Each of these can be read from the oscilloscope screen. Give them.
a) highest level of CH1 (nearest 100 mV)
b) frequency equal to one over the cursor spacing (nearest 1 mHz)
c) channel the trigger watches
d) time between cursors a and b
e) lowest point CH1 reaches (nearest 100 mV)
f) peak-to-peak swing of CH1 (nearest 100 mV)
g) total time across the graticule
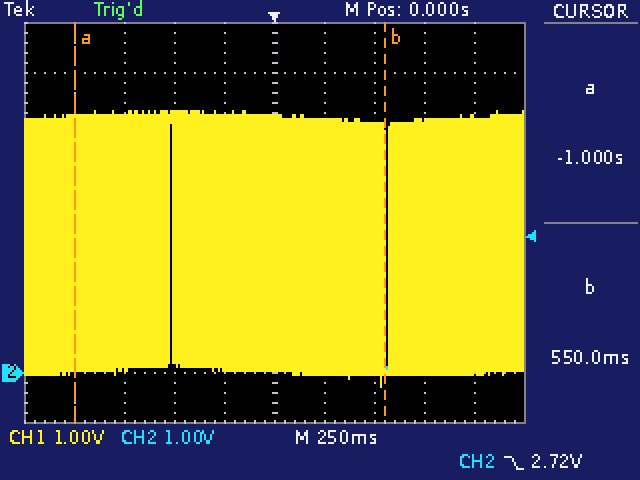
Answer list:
5.2 V
645 mHz
CH2
1.550 s
-300 mV
5.5 V
2.5 s
